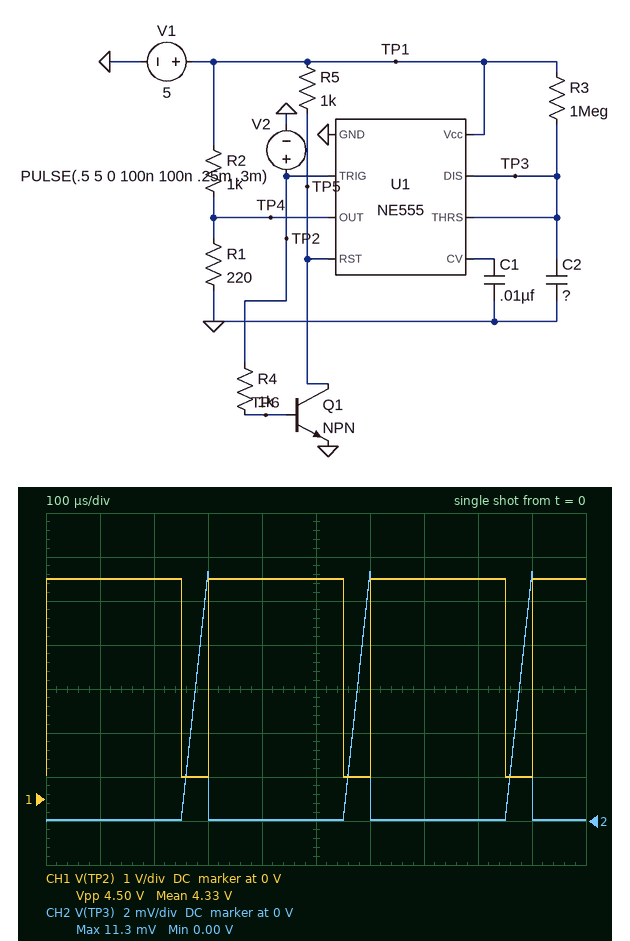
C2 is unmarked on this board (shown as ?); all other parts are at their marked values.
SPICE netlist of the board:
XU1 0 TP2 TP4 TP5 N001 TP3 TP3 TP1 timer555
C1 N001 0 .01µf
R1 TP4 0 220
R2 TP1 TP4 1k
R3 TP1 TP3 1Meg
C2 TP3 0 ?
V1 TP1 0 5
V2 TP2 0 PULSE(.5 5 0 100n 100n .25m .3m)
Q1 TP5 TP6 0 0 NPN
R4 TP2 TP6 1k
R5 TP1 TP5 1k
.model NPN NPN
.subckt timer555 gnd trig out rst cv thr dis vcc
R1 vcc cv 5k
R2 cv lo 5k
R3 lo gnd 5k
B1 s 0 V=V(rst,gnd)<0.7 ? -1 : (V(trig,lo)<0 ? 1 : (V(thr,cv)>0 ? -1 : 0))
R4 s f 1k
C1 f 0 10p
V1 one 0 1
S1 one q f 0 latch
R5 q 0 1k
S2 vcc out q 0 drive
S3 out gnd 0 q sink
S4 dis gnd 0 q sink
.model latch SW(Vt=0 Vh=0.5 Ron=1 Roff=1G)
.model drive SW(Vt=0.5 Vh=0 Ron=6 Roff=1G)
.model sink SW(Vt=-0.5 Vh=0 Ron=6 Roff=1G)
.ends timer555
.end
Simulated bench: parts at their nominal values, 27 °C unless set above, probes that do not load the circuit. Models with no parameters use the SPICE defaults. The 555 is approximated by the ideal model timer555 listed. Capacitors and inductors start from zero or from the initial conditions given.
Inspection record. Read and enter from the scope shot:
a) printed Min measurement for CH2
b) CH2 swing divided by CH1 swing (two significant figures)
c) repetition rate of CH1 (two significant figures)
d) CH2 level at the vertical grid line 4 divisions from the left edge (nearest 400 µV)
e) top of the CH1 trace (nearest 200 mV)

0.00 V
0.0025
3.3 kHz
0 V
5.0 V
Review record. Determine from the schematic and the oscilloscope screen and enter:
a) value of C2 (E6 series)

22 nF
